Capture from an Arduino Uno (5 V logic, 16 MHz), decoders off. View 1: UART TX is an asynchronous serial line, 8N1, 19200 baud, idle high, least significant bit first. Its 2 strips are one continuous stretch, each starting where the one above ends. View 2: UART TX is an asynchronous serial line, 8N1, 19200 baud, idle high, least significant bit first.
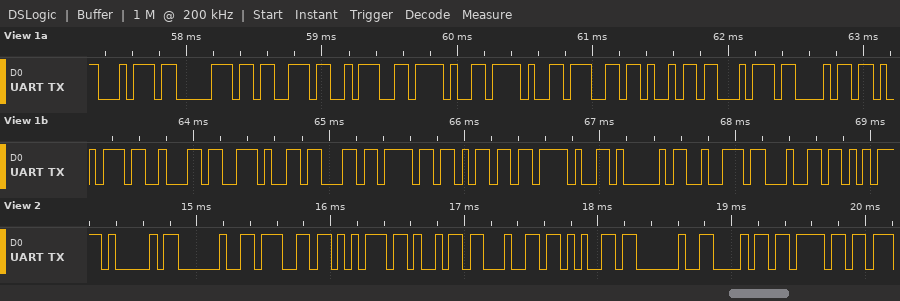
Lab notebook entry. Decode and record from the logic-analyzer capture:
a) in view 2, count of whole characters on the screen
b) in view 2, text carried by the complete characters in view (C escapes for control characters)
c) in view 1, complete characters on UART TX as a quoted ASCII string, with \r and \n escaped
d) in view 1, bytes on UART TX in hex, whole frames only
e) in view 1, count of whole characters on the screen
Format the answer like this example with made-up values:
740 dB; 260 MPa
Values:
10; "A guide ho"; "tps://github.com/Ard"; 74 70 73 3A 2F 2F 67 69 74 68 75 62 2E 63 6F 6D 2F 41 72 64; 20
